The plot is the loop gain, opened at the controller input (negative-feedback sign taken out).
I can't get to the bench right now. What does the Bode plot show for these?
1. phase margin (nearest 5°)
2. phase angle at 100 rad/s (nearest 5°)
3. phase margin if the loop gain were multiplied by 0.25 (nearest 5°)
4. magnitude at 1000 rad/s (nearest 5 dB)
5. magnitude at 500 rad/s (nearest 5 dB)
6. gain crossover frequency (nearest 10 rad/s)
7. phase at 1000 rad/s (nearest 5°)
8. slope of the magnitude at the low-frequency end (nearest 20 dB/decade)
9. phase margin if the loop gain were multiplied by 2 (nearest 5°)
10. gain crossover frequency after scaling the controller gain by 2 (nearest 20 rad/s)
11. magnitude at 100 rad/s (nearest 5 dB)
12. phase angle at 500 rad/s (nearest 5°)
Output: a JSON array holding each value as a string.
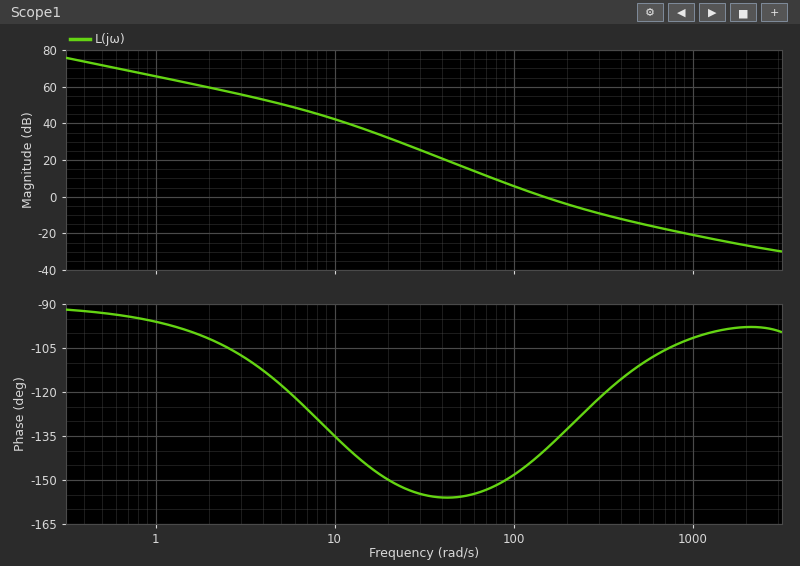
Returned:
["40°", "-150°", "25°", "-20 dB", "-15 dB", "150 rad/s", "-100°", "-20 dB/decade", "50°", "240 rad/s", "5 dB", "-110°"]
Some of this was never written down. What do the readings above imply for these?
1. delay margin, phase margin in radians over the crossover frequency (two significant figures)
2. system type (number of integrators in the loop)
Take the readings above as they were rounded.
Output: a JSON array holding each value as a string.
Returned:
["0.0047 s", "1"]
